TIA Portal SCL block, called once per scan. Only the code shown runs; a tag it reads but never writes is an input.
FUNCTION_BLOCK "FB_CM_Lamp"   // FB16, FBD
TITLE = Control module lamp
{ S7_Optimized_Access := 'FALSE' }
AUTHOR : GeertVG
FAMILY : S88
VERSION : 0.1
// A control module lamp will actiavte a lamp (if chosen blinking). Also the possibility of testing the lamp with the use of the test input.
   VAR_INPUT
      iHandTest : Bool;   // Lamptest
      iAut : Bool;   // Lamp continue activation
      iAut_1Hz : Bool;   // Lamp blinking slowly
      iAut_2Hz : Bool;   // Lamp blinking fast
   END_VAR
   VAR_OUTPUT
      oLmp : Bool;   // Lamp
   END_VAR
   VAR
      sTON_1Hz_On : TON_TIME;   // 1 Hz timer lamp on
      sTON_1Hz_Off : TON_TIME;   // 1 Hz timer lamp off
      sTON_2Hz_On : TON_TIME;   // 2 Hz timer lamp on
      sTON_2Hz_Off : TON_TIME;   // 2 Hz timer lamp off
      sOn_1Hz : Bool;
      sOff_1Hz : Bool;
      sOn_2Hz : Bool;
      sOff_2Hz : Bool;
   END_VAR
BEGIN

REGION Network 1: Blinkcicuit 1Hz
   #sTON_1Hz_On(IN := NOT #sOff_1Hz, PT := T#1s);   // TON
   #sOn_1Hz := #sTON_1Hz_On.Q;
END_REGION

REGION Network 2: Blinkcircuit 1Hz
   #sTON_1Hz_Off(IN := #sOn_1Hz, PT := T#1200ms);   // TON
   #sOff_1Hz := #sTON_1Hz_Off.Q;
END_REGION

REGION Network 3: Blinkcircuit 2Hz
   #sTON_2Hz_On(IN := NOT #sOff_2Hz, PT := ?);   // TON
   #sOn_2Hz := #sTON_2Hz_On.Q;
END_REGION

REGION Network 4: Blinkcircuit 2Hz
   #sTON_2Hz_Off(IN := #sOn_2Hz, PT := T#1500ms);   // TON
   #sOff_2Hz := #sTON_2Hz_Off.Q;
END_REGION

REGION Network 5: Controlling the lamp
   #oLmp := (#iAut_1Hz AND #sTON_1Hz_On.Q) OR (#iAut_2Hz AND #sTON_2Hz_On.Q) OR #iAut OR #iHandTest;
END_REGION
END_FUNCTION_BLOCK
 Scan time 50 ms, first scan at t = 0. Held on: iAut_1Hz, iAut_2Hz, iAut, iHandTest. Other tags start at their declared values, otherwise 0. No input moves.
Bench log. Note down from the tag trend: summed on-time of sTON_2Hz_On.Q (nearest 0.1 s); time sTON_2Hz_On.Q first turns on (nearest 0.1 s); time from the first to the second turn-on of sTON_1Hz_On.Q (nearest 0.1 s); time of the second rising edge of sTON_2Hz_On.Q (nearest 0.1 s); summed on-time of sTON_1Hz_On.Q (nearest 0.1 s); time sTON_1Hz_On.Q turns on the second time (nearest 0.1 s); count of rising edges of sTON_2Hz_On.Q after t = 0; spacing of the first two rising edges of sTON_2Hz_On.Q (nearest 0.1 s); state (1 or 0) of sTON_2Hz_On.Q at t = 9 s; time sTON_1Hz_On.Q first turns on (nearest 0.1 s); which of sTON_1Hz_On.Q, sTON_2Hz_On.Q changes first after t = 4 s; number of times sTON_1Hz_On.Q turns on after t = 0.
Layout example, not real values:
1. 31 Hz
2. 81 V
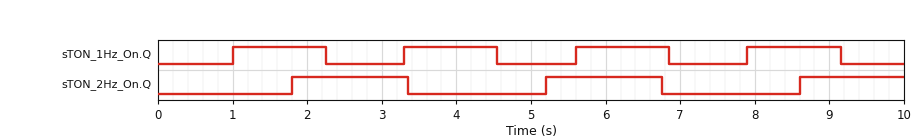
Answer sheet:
1. 4.5 s
2. 1.8 s
3. 2.3 s
4. 5.2 s
5. 5.0 s
6. 3.3 s
7. 3
8. 3.4 s
9. 1
10. 1.0 s
11. sTON_1Hz_On.Q
12. 4
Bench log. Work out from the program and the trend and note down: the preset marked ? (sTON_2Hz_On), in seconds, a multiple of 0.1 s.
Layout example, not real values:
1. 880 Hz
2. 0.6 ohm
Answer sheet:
1. 1.8 s
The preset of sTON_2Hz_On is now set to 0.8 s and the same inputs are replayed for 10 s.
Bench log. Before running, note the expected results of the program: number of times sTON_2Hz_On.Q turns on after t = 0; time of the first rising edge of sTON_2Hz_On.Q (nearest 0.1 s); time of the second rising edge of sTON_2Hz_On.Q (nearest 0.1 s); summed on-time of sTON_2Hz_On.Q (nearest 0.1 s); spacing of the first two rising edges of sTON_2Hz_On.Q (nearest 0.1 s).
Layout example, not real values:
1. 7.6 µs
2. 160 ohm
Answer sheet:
1. 4
2. 0.8 s
3. 3.2 s
4. 6.2 s
5. 2.4 s
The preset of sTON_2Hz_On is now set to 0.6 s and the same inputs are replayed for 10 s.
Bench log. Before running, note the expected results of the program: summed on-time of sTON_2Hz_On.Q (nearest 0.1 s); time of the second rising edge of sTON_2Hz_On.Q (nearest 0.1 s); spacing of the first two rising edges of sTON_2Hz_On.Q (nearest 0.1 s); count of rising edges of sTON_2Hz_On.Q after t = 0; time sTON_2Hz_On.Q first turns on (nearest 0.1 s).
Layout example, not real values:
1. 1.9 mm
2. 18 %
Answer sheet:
1. 6.8 s
2. 2.8 s
3. 2.2 s
4. 5
5. 0.6 s
